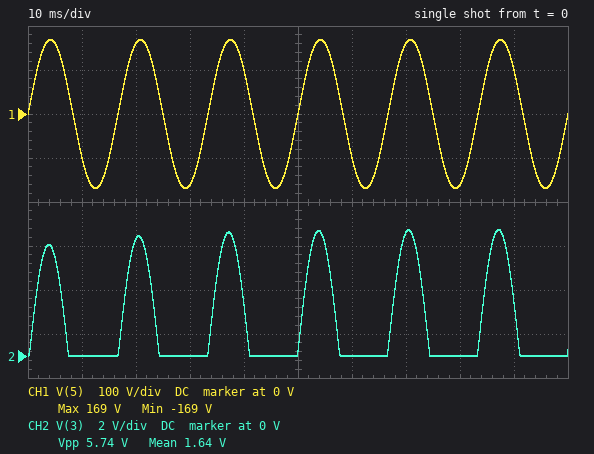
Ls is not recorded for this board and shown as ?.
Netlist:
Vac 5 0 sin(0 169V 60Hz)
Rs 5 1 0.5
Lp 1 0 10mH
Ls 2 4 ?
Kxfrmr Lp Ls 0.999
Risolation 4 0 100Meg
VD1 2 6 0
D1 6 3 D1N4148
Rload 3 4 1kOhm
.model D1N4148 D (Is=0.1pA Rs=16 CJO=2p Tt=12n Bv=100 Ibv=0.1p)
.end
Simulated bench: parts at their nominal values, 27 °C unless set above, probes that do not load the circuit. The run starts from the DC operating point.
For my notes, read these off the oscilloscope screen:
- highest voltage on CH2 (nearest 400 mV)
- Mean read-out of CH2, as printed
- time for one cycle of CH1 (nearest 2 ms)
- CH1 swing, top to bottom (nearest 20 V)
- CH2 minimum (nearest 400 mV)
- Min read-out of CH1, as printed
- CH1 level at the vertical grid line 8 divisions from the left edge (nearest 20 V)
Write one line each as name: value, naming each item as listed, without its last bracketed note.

highest voltage on CH2: 5.6 V
Mean read-out of CH2, as printed: 1.64 V
time for one cycle of CH1: 16 ms
CH1 swing, top to bottom: 340 V
CH2 minimum: 0 V
Min read-out of CH1, as printed: -169 V
CH1 level at the vertical grid line 8 divisions from the left edge: -160 V
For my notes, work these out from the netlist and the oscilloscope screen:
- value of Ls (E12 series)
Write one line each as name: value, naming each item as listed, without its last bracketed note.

value of Ls: 15 µH
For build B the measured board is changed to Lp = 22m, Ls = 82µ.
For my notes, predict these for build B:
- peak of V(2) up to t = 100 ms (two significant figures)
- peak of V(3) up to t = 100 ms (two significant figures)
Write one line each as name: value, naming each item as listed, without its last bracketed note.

peak of V(2) up to t = 100 ms: 10 V
peak of V(3) up to t = 100 ms: 9.4 V
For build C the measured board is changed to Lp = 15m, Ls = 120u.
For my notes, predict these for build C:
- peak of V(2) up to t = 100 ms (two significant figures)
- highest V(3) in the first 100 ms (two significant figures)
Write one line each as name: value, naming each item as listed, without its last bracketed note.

peak of V(2) up to t = 100 ms: 15 V
highest V(3) in the first 100 ms: 14 V
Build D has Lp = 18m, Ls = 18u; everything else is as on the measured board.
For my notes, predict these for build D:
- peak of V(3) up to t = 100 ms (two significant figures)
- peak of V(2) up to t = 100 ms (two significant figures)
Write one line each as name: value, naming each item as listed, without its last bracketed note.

peak of V(3) up to t = 100 ms: 4.6 V
peak of V(2) up to t = 100 ms: 5.3 V
